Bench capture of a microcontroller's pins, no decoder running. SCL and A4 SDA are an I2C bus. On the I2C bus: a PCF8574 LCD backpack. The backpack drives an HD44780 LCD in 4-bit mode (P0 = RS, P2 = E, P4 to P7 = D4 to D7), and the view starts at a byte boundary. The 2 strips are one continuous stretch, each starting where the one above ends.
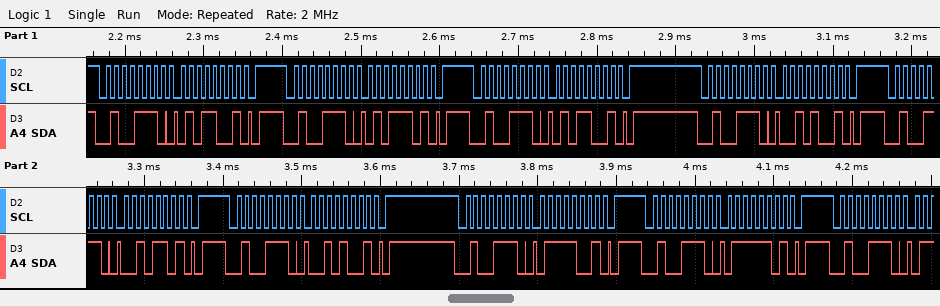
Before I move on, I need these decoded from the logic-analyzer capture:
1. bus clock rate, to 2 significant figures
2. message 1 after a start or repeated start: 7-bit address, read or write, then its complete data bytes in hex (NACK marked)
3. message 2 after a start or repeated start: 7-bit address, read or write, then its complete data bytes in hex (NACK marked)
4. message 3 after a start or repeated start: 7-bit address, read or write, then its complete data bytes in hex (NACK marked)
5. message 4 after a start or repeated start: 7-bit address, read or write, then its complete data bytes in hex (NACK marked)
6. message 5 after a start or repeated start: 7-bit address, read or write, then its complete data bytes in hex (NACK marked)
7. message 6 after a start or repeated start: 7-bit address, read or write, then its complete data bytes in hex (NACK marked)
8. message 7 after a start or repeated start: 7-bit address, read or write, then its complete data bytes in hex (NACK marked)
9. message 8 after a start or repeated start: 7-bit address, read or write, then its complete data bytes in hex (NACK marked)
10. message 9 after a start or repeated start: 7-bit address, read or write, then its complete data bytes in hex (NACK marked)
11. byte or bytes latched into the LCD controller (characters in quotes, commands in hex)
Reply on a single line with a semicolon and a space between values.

100 kHz; 0x27 write: 59; 0x27 write: 5D; 0x27 write: 59; 0x27 write: 29; 0x27 write: 2D; 0x27 write: 29; 0x27 write: 79; 0x27 write: 7D; 0x27 write; 'R'
